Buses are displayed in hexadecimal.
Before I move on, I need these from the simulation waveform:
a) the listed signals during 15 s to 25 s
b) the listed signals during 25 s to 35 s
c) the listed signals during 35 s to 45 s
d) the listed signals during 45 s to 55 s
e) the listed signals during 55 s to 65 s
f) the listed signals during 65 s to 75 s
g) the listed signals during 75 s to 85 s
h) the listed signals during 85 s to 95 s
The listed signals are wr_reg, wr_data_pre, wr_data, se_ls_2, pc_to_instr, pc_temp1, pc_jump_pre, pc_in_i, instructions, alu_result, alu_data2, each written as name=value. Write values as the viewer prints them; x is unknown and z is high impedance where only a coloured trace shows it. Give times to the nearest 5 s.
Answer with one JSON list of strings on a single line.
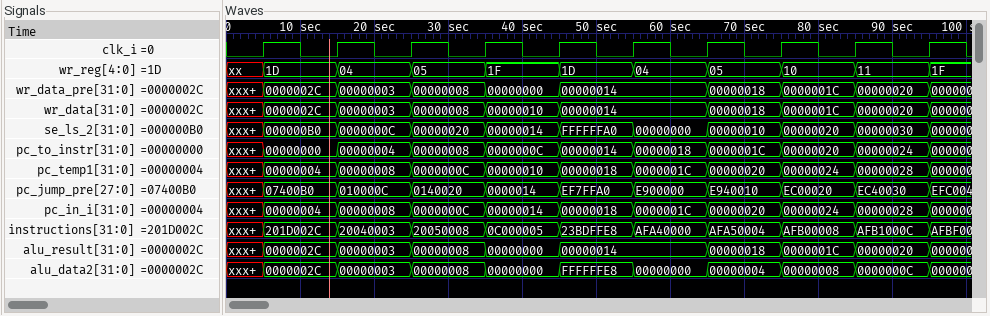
["wr_reg=04, wr_data_pre=00000003, wr_data=00000003, se_ls_2=0000000C, pc_to_instr=00000004, pc_temp1=00000008, pc_jump_pre=010000C, pc_in_i=00000008, instructions=20040003, alu_result=00000003, alu_data2=00000003", "wr_reg=05, wr_data_pre=00000008, wr_data=00000008, se_ls_2=00000020, pc_to_instr=00000008, pc_temp1=0000000C, pc_jump_pre=0140020, pc_in_i=0000000C, instructions=20050008, alu_result=00000008, alu_data2=00000008", "wr_reg=1F, wr_data_pre=00000000, wr_data=00000010, se_ls_2=00000014, pc_to_instr=0000000C, pc_temp1=00000010, pc_jump_pre=0000014, pc_in_i=00000014, instructions=0C000005, alu_result=00000000, alu_data2=00000000", "wr_reg=1D, wr_data_pre=00000014, wr_data=00000014, se_ls_2=FFFFFFA0, pc_to_instr=00000014, pc_temp1=00000018, pc_jump_pre=EF7FFA0, pc_in_i=00000018, instructions=23BDFFE8, alu_result=00000014, alu_data2=FFFFFFE8", "wr_reg=04, wr_data_pre=00000014, wr_data=00000014, se_ls_2=00000000, pc_to_instr=00000018, pc_temp1=0000001C, pc_jump_pre=E900000, pc_in_i=0000001C, instructions=AFA40000, alu_result=00000014, alu_data2=00000000", "wr_reg=05, wr_data_pre=00000018, wr_data=00000018, se_ls_2=00000010, pc_to_instr=0000001C, pc_temp1=00000020, pc_jump_pre=E940010, pc_in_i=00000020, instructions=AFA50004, alu_result=00000018, alu_data2=00000004", "wr_reg=10, wr_data_pre=0000001C, wr_data=0000001C, se_ls_2=00000020, pc_to_instr=00000020, pc_temp1=00000024, pc_jump_pre=EC00020, pc_in_i=00000024, instructions=AFB00008, alu_result=0000001C, alu_data2=00000008", "wr_reg=11, wr_data_pre=00000020, wr_data=00000020, se_ls_2=00000030, pc_to_instr=00000024, pc_temp1=00000028, pc_jump_pre=EC40030, pc_in_i=00000028, instructions=AFB1000C, alu_result=00000020, alu_data2=0000000C"]
